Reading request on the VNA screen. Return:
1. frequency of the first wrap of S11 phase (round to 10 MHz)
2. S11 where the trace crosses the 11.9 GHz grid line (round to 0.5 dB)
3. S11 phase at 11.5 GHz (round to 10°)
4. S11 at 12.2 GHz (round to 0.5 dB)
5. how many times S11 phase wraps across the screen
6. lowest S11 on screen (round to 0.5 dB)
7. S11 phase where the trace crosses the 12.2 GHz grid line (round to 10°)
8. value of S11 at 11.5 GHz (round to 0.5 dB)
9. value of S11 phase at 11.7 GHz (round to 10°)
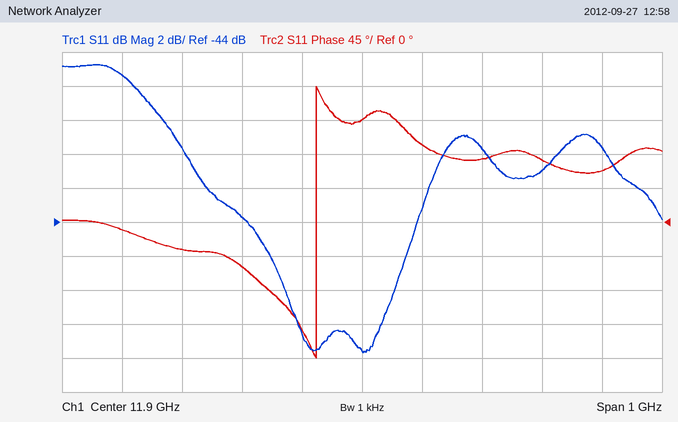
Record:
11.82 GHz
-51.5 dB
-10°
-41.0 dB
1
-51.5 dB
80°
-35.5 dB
-60°
